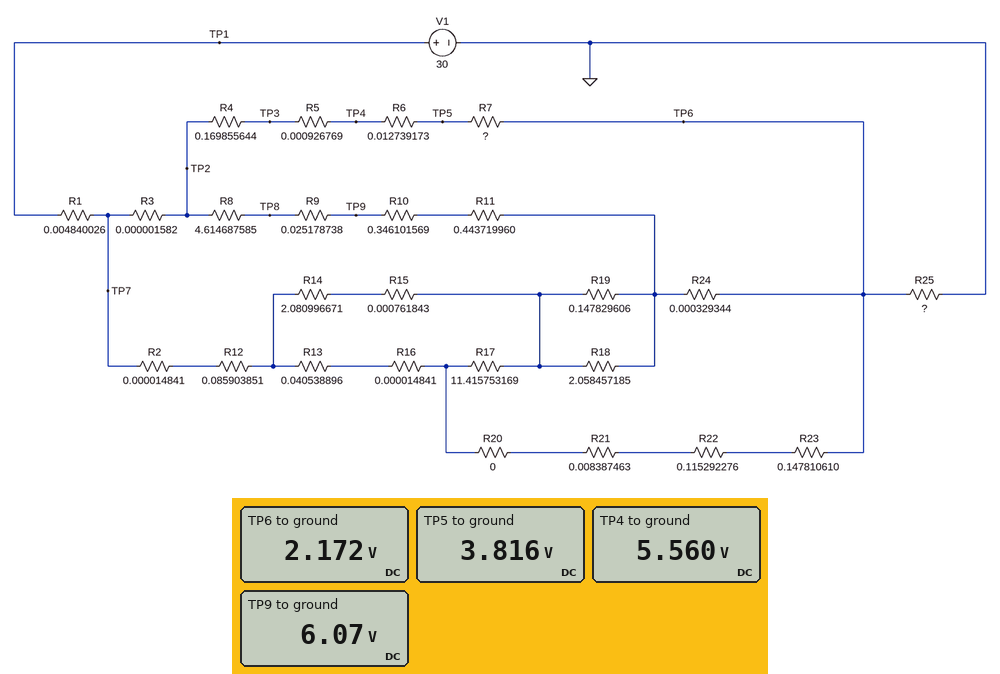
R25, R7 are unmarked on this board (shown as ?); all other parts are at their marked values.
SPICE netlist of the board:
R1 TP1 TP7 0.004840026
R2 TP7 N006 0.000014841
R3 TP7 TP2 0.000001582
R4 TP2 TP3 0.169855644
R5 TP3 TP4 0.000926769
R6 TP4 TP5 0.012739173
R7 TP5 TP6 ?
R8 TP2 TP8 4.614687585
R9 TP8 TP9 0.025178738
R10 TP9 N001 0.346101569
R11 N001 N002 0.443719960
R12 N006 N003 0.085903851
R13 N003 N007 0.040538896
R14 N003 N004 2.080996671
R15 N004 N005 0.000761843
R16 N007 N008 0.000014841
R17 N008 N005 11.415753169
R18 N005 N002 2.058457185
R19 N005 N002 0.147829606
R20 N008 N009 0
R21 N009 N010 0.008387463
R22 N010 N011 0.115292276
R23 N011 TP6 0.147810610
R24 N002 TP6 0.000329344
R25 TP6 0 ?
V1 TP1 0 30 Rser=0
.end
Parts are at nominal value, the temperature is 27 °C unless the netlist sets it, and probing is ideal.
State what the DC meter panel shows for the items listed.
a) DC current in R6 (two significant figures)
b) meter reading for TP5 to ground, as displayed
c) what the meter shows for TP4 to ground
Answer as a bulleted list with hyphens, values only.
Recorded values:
- 140 A
- 3.816 V
- 5.560 V
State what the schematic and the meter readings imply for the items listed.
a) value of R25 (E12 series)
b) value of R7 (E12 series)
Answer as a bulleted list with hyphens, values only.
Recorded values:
- 0.01 Ω
- 0.012 Ω
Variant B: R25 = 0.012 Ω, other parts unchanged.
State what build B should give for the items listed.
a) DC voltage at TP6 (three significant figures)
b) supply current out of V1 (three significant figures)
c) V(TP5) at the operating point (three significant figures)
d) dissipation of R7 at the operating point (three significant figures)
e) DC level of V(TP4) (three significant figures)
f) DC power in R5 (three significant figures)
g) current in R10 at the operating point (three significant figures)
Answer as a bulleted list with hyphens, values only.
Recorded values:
- 2.57 V
- 214 A
- 4.19 V
- 219 W
- 5.91 V
- 16.9 W
- 4.86 A
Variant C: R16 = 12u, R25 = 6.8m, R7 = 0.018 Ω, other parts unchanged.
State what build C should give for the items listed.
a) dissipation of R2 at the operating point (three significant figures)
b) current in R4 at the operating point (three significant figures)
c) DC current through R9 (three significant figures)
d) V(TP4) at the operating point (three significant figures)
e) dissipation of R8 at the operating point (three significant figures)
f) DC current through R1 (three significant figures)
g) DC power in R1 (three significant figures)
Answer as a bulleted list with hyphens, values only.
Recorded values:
- 88.6 mW
- 136 A
- 5.06 A
- 5.67 V
- 118 W
- 219 A
- 231 W
